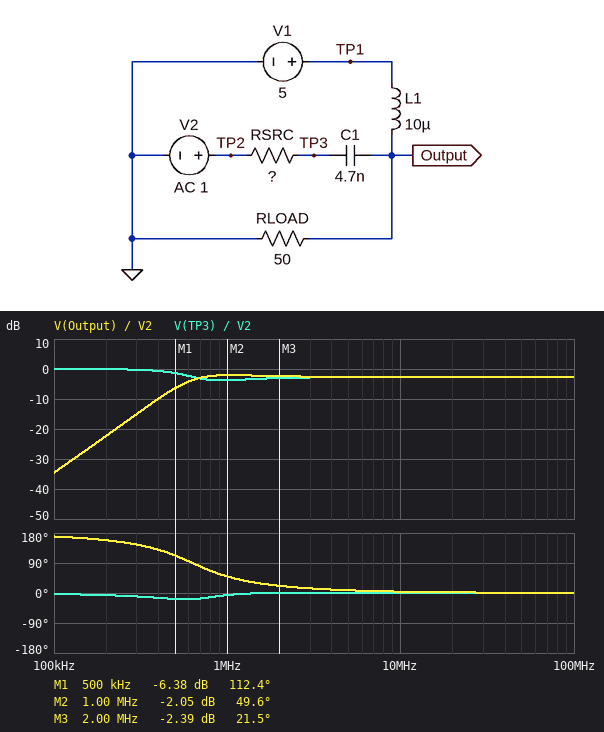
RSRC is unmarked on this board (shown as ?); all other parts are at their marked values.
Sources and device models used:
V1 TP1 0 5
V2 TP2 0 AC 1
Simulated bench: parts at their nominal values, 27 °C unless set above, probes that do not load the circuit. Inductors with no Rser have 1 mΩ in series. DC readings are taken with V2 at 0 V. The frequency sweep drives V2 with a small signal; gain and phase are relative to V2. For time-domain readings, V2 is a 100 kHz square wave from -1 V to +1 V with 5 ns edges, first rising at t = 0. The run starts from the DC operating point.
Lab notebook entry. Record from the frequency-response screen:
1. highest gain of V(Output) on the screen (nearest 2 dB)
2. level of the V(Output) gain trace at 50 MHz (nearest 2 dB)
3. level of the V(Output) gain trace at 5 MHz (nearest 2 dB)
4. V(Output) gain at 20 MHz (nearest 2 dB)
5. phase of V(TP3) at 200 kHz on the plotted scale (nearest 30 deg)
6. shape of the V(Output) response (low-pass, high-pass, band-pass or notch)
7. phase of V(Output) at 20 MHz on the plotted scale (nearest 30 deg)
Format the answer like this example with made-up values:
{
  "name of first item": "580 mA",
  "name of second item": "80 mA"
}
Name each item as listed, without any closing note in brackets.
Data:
{
  "highest gain of V(Output) on the screen": "-2 dB",
  "level of the V(Output) gain trace at 50 MHz": "-2 dB",
  "level of the V(Output) gain trace at 5 MHz": "-2 dB",
  "V(Output) gain at 20 MHz": "-2 dB",
  "phase of V(TP3) at 200 kHz on the plotted scale": "0 deg",
  "shape of the V(Output) response": "high-pass",
  "phase of V(Output) at 20 MHz on the plotted scale": "0 deg"
}
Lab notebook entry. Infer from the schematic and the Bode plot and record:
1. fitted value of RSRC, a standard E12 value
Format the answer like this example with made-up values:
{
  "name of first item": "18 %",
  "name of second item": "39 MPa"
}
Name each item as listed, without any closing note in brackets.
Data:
{
  "fitted value of RSRC, a standard E12 value": "18 Ω"
}
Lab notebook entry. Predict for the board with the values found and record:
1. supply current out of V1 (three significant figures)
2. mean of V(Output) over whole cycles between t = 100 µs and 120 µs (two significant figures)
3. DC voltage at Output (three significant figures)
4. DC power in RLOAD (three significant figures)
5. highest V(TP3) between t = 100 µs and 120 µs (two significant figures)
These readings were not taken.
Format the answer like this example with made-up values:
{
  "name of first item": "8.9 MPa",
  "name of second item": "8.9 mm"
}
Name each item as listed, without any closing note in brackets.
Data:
{
  "supply current out of V1": "100 mA",
  "mean of V(Output) over whole cycles between t = 100 µs and 120 µs": "5.0 V",
  "DC voltage at Output": "5.00 V",
  "DC power in RLOAD": "500 mW",
  "highest V(TP3) between t = 100 µs and 120 µs": "1.1 V"
}
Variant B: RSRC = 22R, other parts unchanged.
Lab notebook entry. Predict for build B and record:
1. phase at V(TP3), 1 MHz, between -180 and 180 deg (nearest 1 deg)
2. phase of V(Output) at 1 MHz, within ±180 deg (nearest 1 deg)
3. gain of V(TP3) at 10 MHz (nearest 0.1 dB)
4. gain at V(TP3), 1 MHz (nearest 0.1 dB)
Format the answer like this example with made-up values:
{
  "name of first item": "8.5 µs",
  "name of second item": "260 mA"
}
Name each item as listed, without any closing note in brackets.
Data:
{
  "phase at V(TP3), 1 MHz, between -180 and 180 deg": "-7 deg",
  "phase of V(Output) at 1 MHz, within ±180 deg": "49 deg",
  "gain of V(TP3) at 10 MHz": "-3.2 dB",
  "gain at V(TP3), 1 MHz": "-4.4 dB"
}
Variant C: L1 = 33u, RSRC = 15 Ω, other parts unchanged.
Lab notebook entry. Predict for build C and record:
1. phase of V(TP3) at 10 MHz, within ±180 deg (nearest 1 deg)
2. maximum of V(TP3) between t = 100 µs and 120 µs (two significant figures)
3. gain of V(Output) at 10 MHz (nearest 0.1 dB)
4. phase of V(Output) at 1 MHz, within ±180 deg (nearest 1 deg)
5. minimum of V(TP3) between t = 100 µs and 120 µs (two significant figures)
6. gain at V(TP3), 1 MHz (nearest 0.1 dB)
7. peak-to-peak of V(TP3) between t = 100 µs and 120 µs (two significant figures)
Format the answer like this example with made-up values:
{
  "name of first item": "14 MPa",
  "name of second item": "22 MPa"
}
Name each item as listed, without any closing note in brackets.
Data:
{
  "phase of V(TP3) at 10 MHz, within ±180 deg": "-1 deg",
  "maximum of V(TP3) between t = 100 µs and 120 µs": "1.0 V",
  "gain of V(Output) at 10 MHz": "-2.3 dB",
  "phase of V(Output) at 1 MHz, within ±180 deg": "33 deg",
  "minimum of V(TP3) between t = 100 µs and 120 µs": "-1.0 V",
  "gain at V(TP3), 1 MHz": "-2.0 dB",
  "peak-to-peak of V(TP3) between t = 100 µs and 120 µs": "2.0 V"
}
